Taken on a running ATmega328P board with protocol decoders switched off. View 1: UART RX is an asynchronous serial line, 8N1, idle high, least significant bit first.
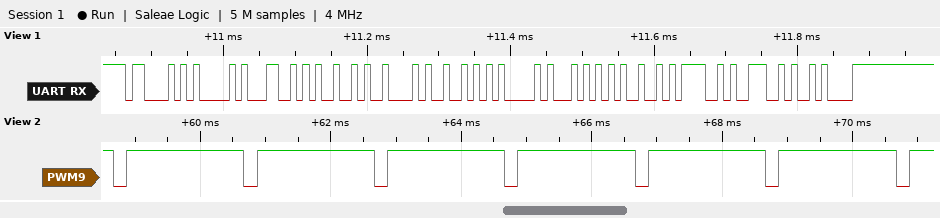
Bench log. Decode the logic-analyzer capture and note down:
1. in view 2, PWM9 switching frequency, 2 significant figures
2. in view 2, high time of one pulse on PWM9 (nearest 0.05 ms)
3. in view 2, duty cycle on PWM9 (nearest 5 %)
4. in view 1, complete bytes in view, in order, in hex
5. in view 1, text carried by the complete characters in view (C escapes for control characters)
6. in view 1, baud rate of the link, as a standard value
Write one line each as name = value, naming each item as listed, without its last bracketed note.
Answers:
in view 2, PWM9 switching frequency, 2 significant figures = 500 Hz
in view 2, high time of one pulse on PWM9 = 1.80 ms
in view 2, duty cycle on PWM9 = 90 %
in view 1, complete bytes in view, in order, in hex = 43 41 4C 49 42 52 41 54 49 4F 4E 0A
in view 1, text carried by the complete characters in view = "CALIBRATION\n"
in view 1, baud rate of the link, as a standard value = 115200 baud
